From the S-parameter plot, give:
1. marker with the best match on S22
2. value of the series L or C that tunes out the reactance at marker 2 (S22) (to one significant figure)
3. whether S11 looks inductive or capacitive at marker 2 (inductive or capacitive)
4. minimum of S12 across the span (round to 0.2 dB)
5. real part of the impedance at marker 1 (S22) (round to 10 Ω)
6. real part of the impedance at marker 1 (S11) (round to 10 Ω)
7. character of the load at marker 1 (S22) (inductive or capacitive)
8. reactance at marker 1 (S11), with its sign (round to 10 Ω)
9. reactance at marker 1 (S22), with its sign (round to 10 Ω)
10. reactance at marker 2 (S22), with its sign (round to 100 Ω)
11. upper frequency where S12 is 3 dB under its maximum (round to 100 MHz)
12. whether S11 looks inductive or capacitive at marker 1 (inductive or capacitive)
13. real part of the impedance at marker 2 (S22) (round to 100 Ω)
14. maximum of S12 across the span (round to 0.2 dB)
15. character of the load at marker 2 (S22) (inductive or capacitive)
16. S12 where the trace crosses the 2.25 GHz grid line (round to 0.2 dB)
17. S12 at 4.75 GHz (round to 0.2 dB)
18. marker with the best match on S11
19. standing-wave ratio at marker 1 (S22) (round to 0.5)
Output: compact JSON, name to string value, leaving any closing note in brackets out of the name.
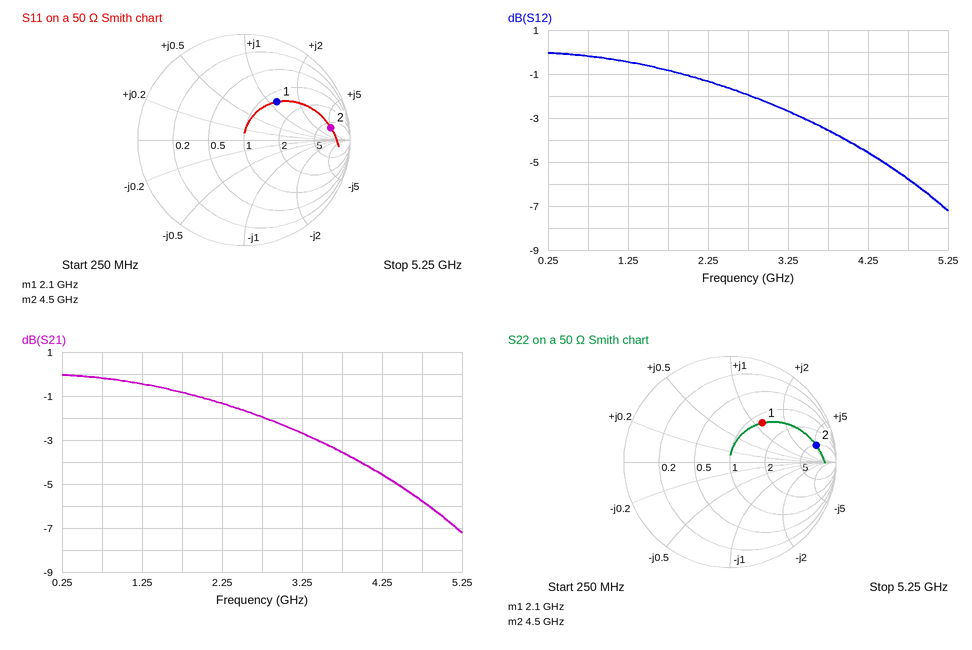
{"marker with the best match on S22": "marker 1", "value of the series L or C that tunes out the reactance at marker 2 (S22)": "100 fF", "whether S11 looks inductive or capacitive at marker 2": "inductive", "minimum of S12 across the span": "-7.2 dB", "real part of the impedance at marker 1 (S22)": "60 Ω", "real part of the impedance at marker 1 (S11)": "60 Ω", "character of the load at marker 1 (S22)": "inductive", "reactance at marker 1 (S11), with its sign": "+60 Ω", "reactance at marker 1 (S22), with its sign": "+60 Ω", "reactance at marker 2 (S22), with its sign": "+300 Ω", "upper frequency where S12 is 3 dB under its maximum": "3.5 GHz", "whether S11 looks inductive or capacitive at marker 1": "inductive", "real part of the impedance at marker 2 (S22)": "300 Ω", "maximum of S12 across the span": "0.0 dB", "character of the load at marker 2 (S22)": "inductive", "S12 where the trace crosses the 2.25 GHz grid line": "-1.4 dB", "S12 at 4.75 GHz": "-5.8 dB", "marker with the best match on S11": "marker 1", "standing-wave ratio at marker 1 (S22)": "3.0"}
